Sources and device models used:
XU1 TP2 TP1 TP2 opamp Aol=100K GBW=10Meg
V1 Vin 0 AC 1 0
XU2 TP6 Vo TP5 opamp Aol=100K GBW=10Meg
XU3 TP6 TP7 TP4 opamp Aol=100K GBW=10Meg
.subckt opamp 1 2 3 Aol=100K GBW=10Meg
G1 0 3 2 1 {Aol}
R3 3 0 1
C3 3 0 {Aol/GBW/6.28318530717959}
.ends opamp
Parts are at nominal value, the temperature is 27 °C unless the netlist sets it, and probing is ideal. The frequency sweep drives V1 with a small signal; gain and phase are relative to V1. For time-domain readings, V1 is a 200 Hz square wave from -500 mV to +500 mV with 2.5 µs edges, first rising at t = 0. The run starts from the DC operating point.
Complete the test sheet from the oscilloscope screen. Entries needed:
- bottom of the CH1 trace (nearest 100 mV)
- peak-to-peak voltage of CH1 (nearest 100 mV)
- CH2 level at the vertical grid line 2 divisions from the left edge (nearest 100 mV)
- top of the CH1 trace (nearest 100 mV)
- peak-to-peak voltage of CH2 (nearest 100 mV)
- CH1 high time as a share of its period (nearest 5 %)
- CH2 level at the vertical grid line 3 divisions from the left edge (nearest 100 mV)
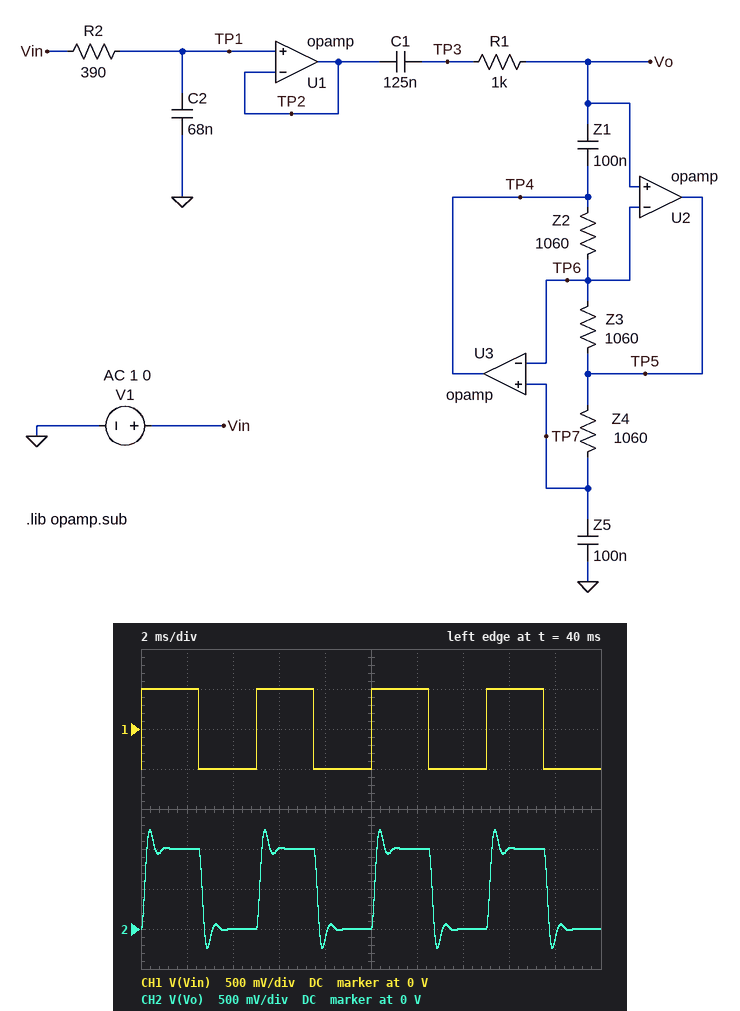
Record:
-500 mV
1.0 V
0 V
500 mV
1.5 V
50 %
1.0 V
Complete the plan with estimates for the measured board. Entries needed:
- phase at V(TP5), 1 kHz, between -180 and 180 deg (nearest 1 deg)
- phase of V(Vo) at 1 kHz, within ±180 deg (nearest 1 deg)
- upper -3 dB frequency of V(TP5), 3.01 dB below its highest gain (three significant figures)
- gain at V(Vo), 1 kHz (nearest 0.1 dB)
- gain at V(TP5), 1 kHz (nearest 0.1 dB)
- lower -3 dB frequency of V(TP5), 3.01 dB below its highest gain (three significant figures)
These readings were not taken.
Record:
-18 deg
-52 deg
2.03 kHz
1.9 dB
3.5 dB
670 Hz
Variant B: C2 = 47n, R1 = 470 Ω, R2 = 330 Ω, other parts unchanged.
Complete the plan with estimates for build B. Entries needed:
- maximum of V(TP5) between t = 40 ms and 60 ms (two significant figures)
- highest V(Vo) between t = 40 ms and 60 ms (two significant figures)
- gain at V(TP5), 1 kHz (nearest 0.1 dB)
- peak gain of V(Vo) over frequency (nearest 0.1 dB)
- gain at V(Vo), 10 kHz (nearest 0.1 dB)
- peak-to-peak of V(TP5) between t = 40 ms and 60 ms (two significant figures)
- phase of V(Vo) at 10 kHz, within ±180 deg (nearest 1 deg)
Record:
1.3 V
1.1 V
1.9 dB
0.3 dB
-28.8 dB
1.7 V
152 deg
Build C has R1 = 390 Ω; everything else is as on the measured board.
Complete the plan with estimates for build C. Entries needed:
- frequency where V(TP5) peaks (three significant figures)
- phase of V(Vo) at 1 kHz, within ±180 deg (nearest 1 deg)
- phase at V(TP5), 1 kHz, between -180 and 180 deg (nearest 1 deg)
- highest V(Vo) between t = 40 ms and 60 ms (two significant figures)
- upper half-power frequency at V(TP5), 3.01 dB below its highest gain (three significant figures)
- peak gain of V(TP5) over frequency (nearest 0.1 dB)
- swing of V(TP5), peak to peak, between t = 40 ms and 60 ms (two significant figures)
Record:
1.99 kHz
-42 deg
-8 deg
1.1 V
3.62 kHz
3.0 dB
1.6 V
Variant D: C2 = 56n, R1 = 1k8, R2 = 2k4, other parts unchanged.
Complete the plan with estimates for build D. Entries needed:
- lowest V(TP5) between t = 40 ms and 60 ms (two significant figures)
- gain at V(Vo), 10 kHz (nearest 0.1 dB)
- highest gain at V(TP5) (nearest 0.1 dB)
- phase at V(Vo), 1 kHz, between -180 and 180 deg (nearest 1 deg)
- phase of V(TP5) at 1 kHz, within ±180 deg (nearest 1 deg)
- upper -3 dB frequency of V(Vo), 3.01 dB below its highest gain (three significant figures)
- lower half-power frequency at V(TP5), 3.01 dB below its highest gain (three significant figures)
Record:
-310 mV
-56.2 dB
3.9 dB
-105 deg
-72 deg
1.29 kHz
448 Hz
